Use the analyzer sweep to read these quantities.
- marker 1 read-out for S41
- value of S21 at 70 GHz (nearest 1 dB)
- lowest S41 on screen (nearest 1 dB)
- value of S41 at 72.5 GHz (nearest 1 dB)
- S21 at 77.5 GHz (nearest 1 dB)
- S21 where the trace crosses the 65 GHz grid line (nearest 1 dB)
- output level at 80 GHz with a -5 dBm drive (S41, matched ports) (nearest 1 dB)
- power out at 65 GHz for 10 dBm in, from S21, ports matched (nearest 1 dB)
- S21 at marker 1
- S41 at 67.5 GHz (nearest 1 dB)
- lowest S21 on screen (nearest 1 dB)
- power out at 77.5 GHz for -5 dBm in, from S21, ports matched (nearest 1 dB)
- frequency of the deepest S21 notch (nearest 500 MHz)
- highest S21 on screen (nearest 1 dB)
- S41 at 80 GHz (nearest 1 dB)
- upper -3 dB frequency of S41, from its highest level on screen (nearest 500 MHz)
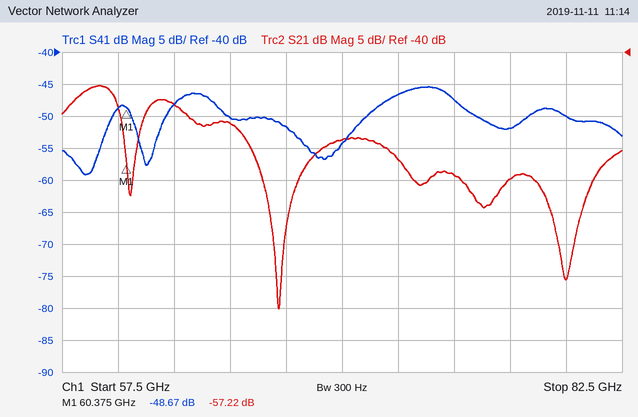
-48.67 dB
-54 dB
-59 dB
-47 dB
-60 dB
-51 dB
-55 dBm
-41 dBm
-57.22 dB
-52 dB
-80 dB
-65 dBm
67.0 GHz
-45 dB
-50 dB
75.5 GHz
